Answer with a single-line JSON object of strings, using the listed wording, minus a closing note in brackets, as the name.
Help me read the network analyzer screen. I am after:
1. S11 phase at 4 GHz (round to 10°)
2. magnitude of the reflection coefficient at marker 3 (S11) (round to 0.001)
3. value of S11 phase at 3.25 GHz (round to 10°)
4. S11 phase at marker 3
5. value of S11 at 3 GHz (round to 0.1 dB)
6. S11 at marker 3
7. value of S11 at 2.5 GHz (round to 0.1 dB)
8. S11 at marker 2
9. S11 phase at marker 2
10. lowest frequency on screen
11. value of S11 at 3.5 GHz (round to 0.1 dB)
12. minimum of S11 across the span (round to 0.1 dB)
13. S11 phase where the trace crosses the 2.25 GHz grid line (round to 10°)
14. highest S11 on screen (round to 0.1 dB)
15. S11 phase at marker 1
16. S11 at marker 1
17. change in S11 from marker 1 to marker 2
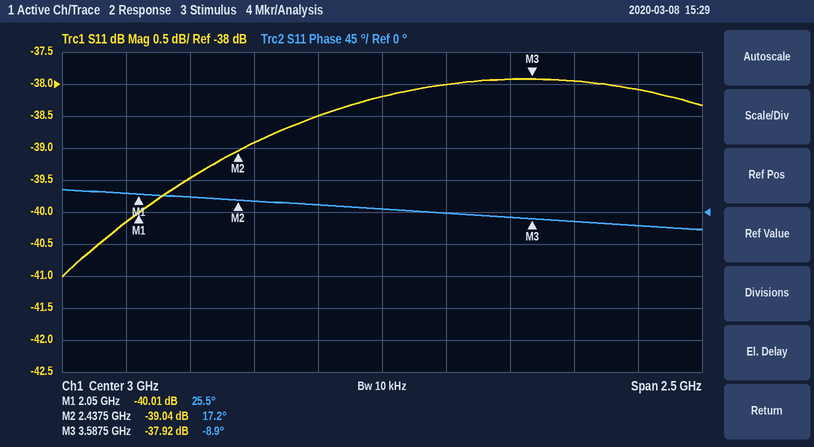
{"S11 phase at 4 GHz": "-20°", "magnitude of the reflection coefficient at marker 3 (S11)": "0.013", "value of S11 phase at 3.25 GHz": "0°", "S11 phase at marker 3": "-8.9°", "value of S11 at 3 GHz": "-38.2 dB", "S11 at marker 3": "-37.92 dB", "value of S11 at 2.5 GHz": "-38.9 dB", "S11 at marker 2": "-39.04 dB", "S11 phase at marker 2": "17.2°", "lowest frequency on screen": "1.75 GHz", "value of S11 at 3.5 GHz": "-37.9 dB", "minimum of S11 across the span": "-41.0 dB", "S11 phase where the trace crosses the 2.25 GHz grid line": "20°", "highest S11 on screen": "-37.9 dB", "S11 phase at marker 1": "25.5°", "S11 at marker 1": "-40.01 dB", "change in S11 from marker 1 to marker 2": "0.97 dB"}
